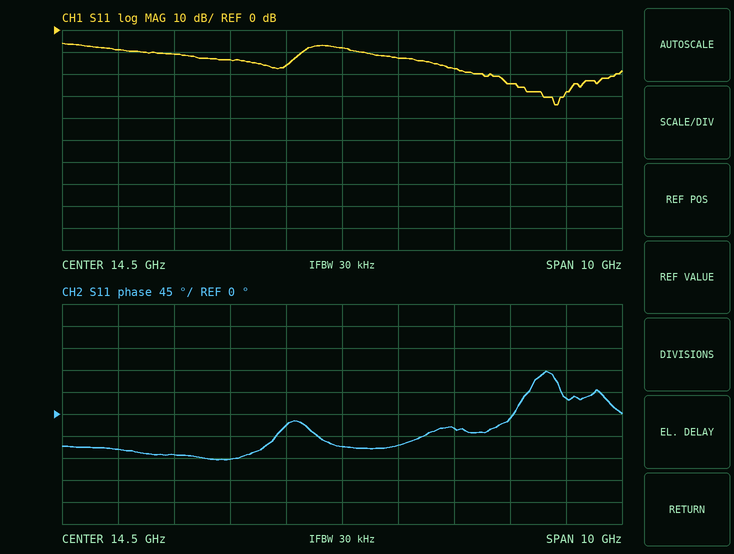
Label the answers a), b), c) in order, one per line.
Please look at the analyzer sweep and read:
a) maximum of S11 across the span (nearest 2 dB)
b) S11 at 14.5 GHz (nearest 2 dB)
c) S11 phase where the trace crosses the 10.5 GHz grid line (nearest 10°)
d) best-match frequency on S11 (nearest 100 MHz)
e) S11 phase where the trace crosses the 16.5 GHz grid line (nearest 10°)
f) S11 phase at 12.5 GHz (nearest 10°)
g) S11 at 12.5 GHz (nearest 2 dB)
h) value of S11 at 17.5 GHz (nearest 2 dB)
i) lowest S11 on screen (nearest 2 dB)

a) -6 dB
b) -8 dB
c) -70°
d) 18.3 GHz
e) -30°
f) -90°
g) -14 dB
h) -24 dB
i) -34 dB
